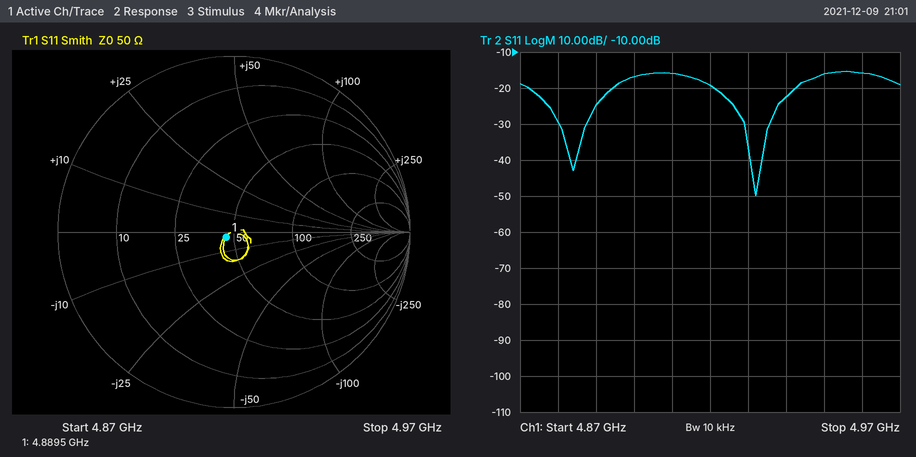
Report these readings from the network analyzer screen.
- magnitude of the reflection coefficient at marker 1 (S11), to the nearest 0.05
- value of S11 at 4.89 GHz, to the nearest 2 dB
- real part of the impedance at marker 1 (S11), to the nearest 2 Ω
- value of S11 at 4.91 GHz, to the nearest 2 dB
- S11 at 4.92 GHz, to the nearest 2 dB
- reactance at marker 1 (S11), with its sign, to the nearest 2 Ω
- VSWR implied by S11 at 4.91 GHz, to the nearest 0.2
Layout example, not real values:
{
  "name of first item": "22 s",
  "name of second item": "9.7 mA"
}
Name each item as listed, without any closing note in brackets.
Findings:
{
  "magnitude of the reflection coefficient at marker 1 (S11), to the nearest 0.05": "0.05",
  "value of S11 at 4.89 GHz, to the nearest 2 dB": "-24 dB",
  "real part of the impedance at marker 1 (S11), to the nearest 2 Ω": "46 Ω",
  "value of S11 at 4.91 GHz, to the nearest 2 dB": "-16 dB",
  "S11 at 4.92 GHz, to the nearest 2 dB": "-20 dB",
  "reactance at marker 1 (S11), with its sign, to the nearest 2 Ω": "-2 Ω",
  "VSWR implied by S11 at 4.91 GHz, to the nearest 0.2": "1.4"
}
